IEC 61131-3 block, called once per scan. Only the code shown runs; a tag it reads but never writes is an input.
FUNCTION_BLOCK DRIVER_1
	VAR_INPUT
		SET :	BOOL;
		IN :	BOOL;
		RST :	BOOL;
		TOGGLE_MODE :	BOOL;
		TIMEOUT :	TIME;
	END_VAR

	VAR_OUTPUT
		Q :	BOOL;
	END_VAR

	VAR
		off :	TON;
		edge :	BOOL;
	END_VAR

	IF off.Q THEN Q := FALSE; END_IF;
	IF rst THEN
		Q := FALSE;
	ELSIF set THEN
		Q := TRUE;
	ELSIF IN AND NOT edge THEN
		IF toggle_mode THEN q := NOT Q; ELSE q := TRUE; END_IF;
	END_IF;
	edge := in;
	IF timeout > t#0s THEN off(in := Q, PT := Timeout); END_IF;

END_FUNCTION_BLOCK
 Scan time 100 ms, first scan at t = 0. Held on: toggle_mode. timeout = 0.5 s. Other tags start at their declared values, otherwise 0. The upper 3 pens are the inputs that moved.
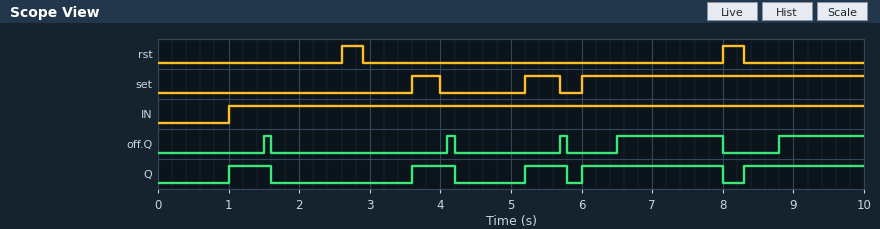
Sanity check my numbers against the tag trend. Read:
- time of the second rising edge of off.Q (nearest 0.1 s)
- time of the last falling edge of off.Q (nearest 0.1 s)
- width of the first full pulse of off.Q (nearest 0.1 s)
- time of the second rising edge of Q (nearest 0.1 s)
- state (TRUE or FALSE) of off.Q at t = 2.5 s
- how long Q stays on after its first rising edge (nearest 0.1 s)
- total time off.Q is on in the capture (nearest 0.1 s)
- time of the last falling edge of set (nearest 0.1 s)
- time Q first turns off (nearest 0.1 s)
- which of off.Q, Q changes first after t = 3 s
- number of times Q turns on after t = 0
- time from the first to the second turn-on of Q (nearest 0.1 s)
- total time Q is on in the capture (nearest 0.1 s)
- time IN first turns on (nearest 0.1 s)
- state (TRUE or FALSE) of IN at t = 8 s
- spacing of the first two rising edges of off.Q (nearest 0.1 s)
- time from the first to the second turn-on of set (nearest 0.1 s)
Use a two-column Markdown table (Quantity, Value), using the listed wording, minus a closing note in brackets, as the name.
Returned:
| Quantity | Value |
|---|---|
| time of the second rising edge of off.Q | 4.1 s |
| time of the last falling edge of off.Q | 8.0 s |
| width of the first full pulse of off.Q | 0.1 s |
| time of the second rising edge of Q | 3.6 s |
| state (TRUE or FALSE) of off.Q at t = 2.5 s | FALSE |
| how long Q stays on after its first rising edge | 0.6 s |
| total time off.Q is on in the capture | 3.0 s |
| time of the last falling edge of set | 5.7 s |
| time Q first turns off | 1.6 s |
| which of off.Q, Q changes first after t = 3 s | Q |
| number of times Q turns on after t = 0 | 5 |
| time from the first to the second turn-on of Q | 2.6 s |
| total time Q is on in the capture | 5.5 s |
| time IN first turns on | 1.0 s |
| state (TRUE or FALSE) of IN at t = 8 s | TRUE |
| spacing of the first two rising edges of off.Q | 2.6 s |
| time from the first to the second turn-on of set | 1.6 s |
